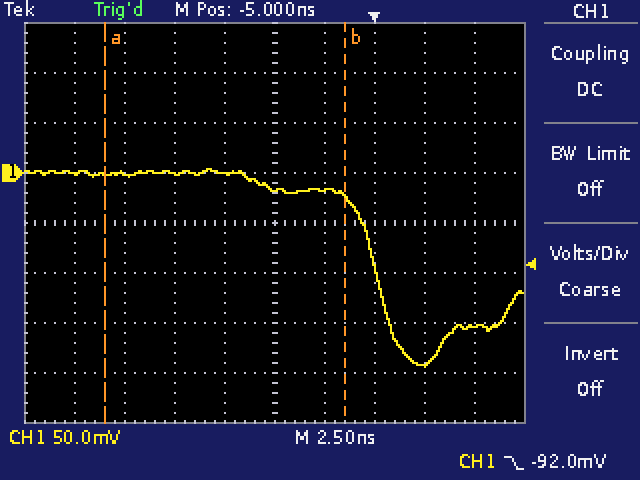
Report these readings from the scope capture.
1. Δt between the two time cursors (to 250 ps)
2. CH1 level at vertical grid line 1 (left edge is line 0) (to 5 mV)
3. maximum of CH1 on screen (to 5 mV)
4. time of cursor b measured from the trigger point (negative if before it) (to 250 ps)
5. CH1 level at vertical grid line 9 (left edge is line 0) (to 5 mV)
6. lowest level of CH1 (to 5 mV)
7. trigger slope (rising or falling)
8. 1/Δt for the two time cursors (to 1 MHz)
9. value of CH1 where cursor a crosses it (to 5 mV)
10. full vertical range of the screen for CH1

12.00 ns
0 mV
5 mV
-1.50 ns
-155 mV
-195 mV
falling
83 MHz
0 mV
400 mV
